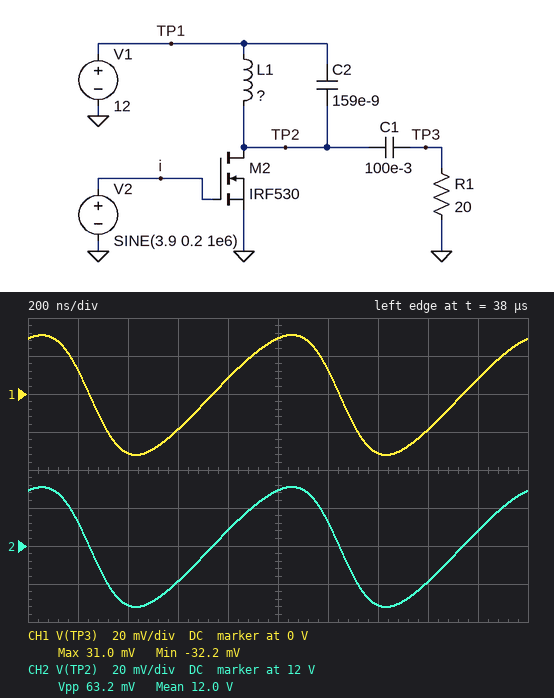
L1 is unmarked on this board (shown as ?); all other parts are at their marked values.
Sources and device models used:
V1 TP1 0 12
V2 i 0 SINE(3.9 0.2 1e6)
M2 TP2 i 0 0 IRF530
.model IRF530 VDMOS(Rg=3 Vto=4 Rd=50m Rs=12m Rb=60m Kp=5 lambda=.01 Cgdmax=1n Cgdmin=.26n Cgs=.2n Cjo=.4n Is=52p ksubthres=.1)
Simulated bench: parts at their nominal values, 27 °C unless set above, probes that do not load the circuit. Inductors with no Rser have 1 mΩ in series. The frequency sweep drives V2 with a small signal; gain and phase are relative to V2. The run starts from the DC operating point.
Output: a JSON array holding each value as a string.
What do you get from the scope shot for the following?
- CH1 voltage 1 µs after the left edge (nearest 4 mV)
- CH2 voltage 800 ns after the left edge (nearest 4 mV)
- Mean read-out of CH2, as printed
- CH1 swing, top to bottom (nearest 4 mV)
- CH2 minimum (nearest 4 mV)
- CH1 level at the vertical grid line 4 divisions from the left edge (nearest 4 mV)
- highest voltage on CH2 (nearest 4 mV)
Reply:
["28 mV", "12.008 V", "12.0 V", "64 mV", "11.968 V", "8 mV", "12.032 V"]
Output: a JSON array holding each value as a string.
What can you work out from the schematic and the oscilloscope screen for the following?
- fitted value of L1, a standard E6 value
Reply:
["470 nH"]
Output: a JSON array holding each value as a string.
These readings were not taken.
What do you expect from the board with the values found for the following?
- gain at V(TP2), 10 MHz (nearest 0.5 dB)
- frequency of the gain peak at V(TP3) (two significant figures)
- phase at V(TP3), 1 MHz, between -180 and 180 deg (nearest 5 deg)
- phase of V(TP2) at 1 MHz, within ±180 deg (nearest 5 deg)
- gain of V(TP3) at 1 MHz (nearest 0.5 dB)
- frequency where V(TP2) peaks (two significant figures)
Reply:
["-46.0 dB", "580 kHz", "90 deg", "90 deg", "-23.0 dB", "580 kHz"]
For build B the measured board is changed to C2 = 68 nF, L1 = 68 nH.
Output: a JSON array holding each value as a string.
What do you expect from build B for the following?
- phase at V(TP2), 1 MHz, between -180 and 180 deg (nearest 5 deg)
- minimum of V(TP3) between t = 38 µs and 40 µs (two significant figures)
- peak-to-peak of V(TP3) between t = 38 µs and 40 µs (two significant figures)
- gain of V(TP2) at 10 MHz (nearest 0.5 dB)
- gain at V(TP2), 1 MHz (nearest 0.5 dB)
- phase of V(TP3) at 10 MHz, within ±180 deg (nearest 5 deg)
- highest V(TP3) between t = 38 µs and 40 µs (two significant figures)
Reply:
["-95 deg", "-37 mV", "79 mV", "-38.0 dB", "-32.0 dB", "65 deg", "42 mV"]
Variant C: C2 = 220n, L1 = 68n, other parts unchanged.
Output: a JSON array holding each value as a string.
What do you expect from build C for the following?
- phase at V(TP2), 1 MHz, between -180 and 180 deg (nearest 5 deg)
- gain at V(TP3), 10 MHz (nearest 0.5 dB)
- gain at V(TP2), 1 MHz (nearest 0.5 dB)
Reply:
["-95 deg", "-48.5 dB", "-26.0 dB"]
